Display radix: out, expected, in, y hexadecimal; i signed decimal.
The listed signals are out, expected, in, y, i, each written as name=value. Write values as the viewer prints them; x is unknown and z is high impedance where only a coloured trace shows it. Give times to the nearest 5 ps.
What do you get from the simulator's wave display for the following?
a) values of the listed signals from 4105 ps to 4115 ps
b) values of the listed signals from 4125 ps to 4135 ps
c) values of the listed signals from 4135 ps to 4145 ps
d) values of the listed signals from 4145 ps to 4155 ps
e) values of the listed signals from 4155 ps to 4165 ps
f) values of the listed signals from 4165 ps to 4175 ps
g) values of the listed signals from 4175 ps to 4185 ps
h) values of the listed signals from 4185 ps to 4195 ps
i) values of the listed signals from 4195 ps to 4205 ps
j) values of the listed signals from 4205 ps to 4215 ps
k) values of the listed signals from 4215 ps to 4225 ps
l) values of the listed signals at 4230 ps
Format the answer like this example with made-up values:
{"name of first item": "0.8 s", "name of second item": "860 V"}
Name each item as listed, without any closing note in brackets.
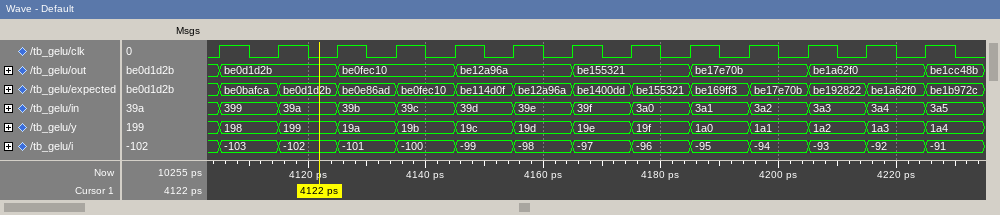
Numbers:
{"values of the listed signals from 4105 ps to 4115 ps": "out=be0d1d2b, expected=be0bafca, in=399, y=198, i=-103", "values of the listed signals from 4125 ps to 4135 ps": "out=be0fec10, expected=be0e86ad, in=39b, y=19a, i=-101", "values of the listed signals from 4135 ps to 4145 ps": "out=be0fec10, expected=be0fec10, in=39c, y=19b, i=-100", "values of the listed signals from 4145 ps to 4155 ps": "out=be12a96a, expected=be114d0f, in=39d, y=19c, i=-99", "values of the listed signals from 4155 ps to 4165 ps": "out=be12a96a, expected=be12a96a, in=39e, y=19d, i=-98", "values of the listed signals from 4165 ps to 4175 ps": "out=be155321, expected=be1400dd, in=39f, y=19e, i=-97", "values of the listed signals from 4175 ps to 4185 ps": "out=be155321, expected=be155321, in=3a0, y=19f, i=-96", "values of the listed signals from 4185 ps to 4195 ps": "out=be17e70b, expected=be169ff3, in=3a1, y=1a0, i=-95", "values of the listed signals from 4195 ps to 4205 ps": "out=be17e70b, expected=be17e70b, in=3a2, y=1a1, i=-94", "values of the listed signals from 4205 ps to 4215 ps": "out=be1a62f0, expected=be192822, in=3a3, y=1a2, i=-93", "values of the listed signals from 4215 ps to 4225 ps": "out=be1a62f0, expected=be1a62f0, in=3a4, y=1a3, i=-92", "values of the listed signals at 4230 ps": "out=be1cc48b, expected=be1b972c, in=3a5, y=1a4, i=-91"}
